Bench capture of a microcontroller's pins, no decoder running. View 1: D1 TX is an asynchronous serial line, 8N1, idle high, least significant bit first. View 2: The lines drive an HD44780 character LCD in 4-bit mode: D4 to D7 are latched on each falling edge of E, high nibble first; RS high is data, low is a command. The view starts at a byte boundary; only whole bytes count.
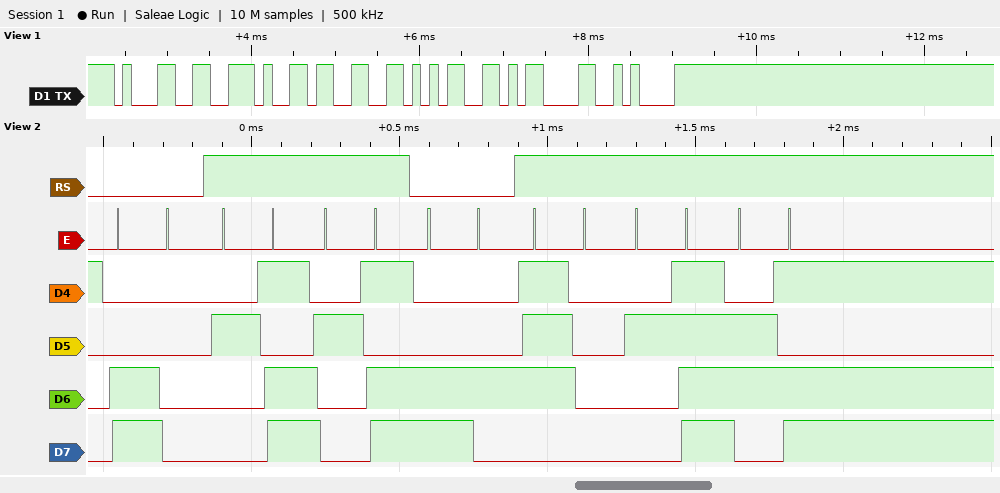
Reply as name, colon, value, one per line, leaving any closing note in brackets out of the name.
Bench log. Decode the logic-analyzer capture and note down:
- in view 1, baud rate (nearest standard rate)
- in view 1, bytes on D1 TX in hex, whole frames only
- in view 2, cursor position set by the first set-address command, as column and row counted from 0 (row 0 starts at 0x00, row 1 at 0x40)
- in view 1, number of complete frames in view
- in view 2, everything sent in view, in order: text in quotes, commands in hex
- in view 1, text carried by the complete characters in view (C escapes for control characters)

in view 1, baud rate: 9600 baud
in view 1, bytes on D1 TX in hex, whole frames only: 31 2E 33 35 0D 0A
in view 2, cursor position set by the first set-address command, as column and row counted from 0: column 0, row 1
in view 1, number of complete frames in view: 6
in view 2, everything sent in view, in order: text in quotes, commands in hex: 0xC0 "--" 0xC4 "p/m"
in view 1, text carried by the complete characters in view: "1.35\r\n"
